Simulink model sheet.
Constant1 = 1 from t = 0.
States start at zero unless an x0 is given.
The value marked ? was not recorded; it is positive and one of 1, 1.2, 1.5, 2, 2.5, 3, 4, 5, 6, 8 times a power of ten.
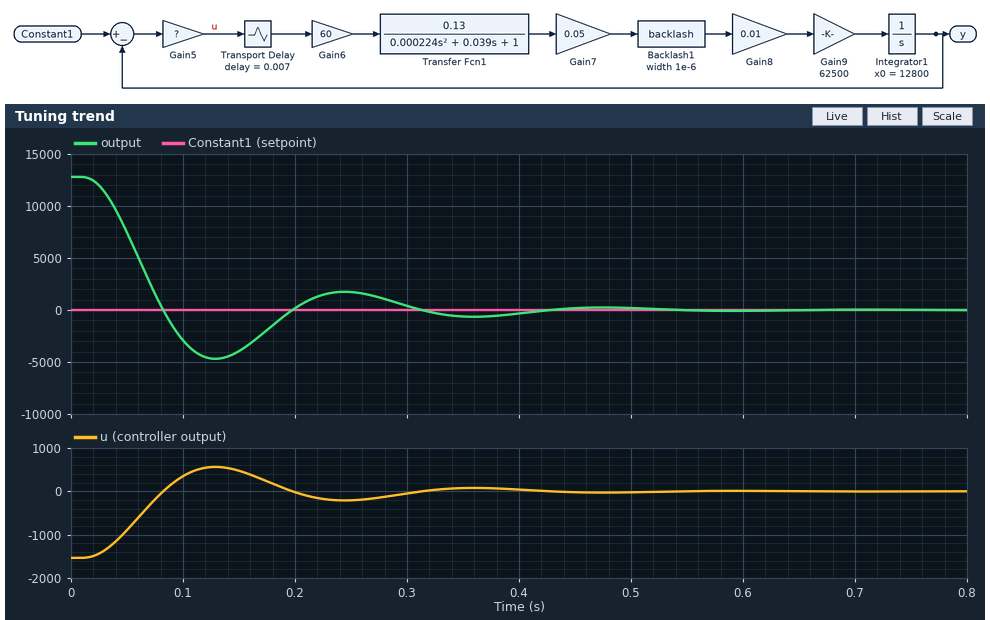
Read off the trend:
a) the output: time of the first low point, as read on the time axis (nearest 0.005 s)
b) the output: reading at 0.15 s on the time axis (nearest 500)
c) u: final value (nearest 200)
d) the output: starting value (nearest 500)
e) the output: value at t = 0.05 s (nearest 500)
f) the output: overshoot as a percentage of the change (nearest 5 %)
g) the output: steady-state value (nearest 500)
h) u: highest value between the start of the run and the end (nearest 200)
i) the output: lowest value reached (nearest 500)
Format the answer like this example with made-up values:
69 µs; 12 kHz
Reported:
0.130 s; -4000; 0; 13000; 7500; 35 %; 0; 600; -4500
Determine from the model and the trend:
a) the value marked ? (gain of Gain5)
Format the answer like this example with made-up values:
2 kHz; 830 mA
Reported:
0.12
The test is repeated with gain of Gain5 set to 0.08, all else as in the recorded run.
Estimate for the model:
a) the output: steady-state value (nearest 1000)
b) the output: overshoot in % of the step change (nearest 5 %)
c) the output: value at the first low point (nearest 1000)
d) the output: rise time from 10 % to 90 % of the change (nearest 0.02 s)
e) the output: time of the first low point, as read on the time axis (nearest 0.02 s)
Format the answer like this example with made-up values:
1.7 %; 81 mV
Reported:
0; 20 %; -3000; 0.06 s; 0.16 s
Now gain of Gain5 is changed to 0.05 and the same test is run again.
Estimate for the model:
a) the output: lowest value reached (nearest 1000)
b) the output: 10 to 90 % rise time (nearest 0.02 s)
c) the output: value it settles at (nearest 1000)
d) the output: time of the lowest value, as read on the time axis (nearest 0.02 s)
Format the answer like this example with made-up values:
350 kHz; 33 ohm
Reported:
-1000; 0.10 s; 0; 0.24 s
